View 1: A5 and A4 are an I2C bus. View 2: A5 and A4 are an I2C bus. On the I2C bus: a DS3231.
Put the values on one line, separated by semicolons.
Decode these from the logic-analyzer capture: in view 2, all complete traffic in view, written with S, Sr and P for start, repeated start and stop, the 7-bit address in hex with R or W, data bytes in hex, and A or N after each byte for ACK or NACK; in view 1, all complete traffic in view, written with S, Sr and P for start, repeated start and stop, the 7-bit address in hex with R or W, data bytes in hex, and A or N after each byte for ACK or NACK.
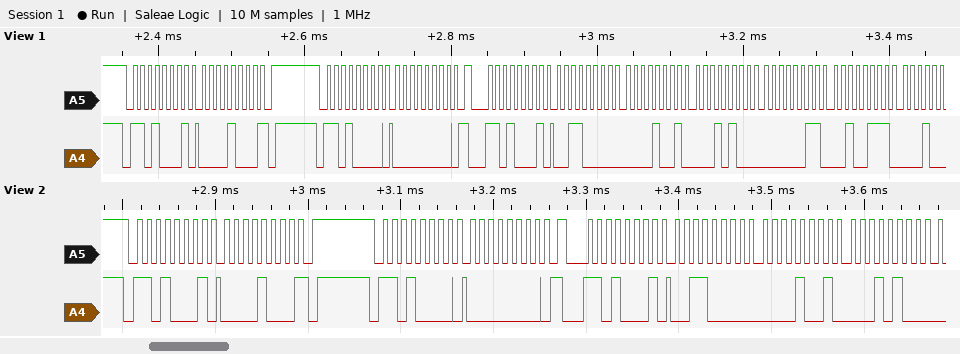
S 68R A 08 N P S 68W A 00 A Sr 68R A 30 A 09 A 14 A; S 68R A 08 N P S 68W A 00 A Sr 68R A 30 A 09 A 14 A 03 A 27 A
